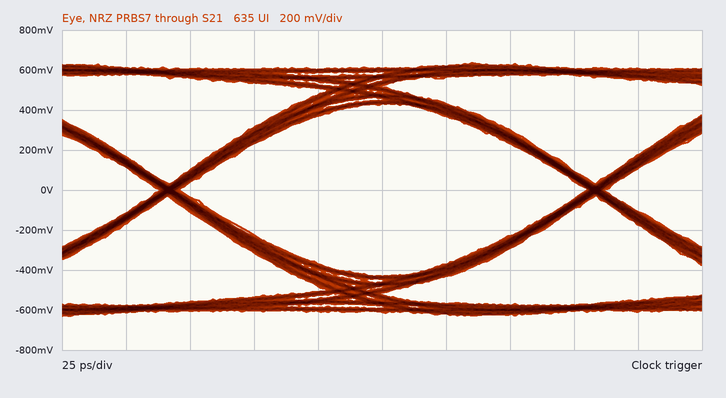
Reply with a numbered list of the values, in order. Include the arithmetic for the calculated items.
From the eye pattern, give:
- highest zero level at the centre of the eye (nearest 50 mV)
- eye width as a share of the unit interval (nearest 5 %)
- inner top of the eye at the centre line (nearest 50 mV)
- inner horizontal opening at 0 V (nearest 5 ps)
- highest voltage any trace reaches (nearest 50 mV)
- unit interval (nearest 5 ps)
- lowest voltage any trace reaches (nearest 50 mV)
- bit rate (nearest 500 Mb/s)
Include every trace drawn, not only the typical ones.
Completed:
1. -450 mV
2. 160 ps / 165 ps ≈ 97.0 %, so 95 % to the nearest 5 %
3. 450 mV
4. 160 ps
5. 650 mV
6. 165 ps
7. -650 mV
8. 6.0 Gb/s
